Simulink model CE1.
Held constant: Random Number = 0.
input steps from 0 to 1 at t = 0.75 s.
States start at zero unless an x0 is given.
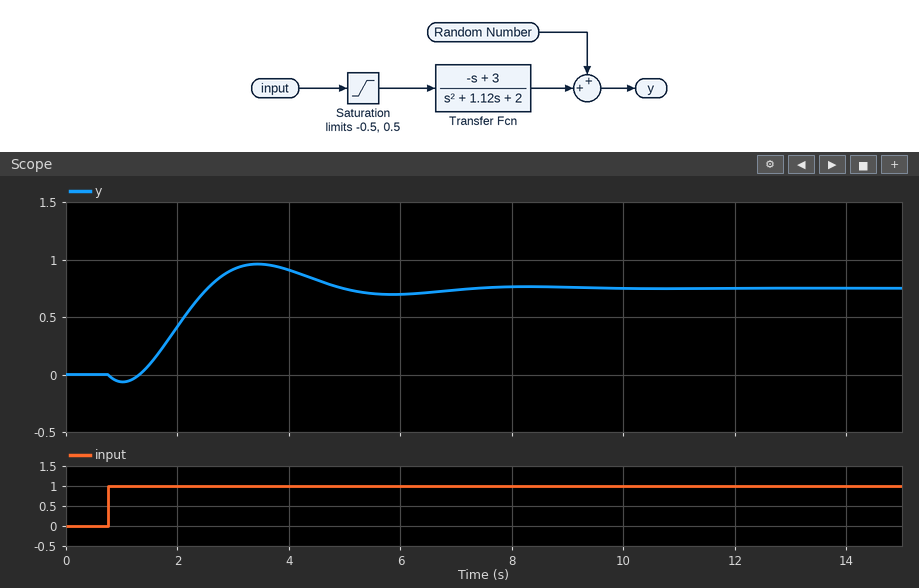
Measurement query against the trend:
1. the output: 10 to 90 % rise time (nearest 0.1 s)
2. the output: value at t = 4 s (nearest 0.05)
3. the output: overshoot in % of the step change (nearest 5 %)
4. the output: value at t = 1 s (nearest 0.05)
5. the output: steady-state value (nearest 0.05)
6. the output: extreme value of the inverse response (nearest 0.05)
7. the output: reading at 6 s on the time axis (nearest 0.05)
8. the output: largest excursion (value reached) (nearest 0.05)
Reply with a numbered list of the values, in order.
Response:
1. 0.9 s
2. 0.90
3. 30 %
4. -0.05
5. 0.75
6. -0.05
7. 0.70
8. 0.95
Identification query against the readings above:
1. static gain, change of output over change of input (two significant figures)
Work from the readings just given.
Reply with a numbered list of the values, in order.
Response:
1. 0.75
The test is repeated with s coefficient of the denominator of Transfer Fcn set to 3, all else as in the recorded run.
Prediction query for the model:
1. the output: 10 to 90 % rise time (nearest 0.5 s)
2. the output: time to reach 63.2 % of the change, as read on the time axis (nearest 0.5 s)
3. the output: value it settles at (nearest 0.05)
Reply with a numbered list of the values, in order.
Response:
1. 2.5 s
2. 2.5 s
3. 0.75
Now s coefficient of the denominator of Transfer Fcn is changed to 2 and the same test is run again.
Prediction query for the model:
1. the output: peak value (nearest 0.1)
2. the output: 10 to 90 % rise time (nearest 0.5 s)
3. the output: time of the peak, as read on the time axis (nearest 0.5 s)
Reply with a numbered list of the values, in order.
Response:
1. 0.8
2. 1.5 s
3. 4.0 s
